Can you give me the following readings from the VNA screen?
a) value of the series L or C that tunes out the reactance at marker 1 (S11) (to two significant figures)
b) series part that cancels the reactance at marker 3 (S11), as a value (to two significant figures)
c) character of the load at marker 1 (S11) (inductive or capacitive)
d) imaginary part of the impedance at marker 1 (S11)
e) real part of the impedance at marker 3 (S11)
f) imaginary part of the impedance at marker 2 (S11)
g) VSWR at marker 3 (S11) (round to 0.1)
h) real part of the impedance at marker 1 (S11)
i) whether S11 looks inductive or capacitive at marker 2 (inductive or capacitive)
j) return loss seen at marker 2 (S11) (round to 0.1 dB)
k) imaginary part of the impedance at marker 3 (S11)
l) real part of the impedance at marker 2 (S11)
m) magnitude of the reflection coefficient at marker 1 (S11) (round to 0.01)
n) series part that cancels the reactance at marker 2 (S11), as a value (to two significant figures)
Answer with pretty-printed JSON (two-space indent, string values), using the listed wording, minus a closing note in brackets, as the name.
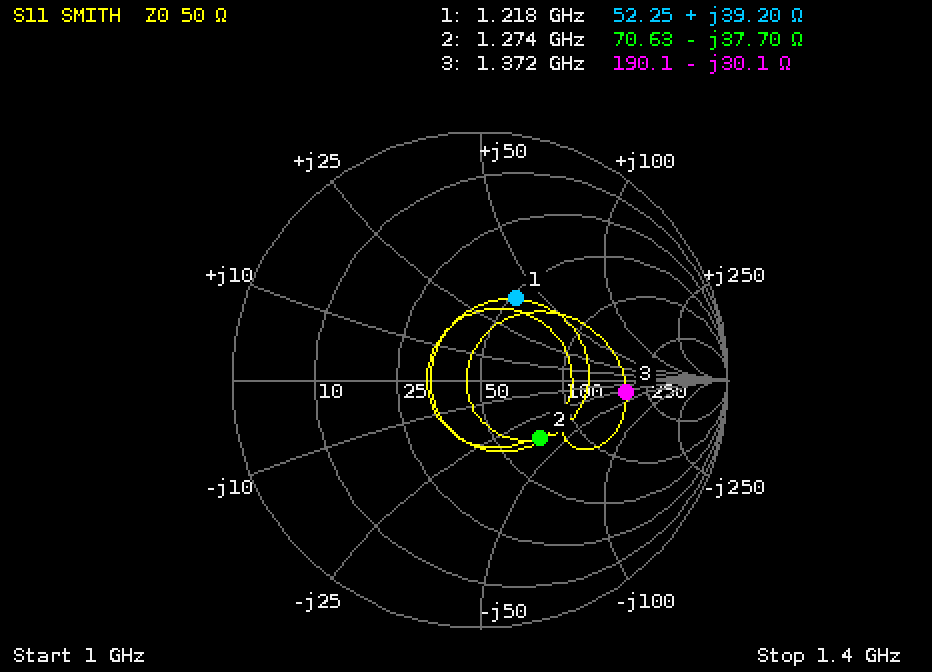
{
  "value of the series L or C that tunes out the reactance at marker 1 (S11)": "3.3 pF",
  "series part that cancels the reactance at marker 3 (S11), as a value": "3.5 nH",
  "character of the load at marker 1 (S11)": "inductive",
  "imaginary part of the impedance at marker 1": "+39.20 Ω",
  "real part of the impedance at marker 3": "190.1 Ω",
  "imaginary part of the impedance at marker 2": "-37.70 Ω",
  "VSWR at marker 3 (S11)": "3.9",
  "real part of the impedance at marker 1": "52.25 Ω",
  "whether S11 looks inductive or capacitive at marker 2": "capacitive",
  "return loss seen at marker 2 (S11)": "9.4 dB",
  "imaginary part of the impedance at marker 3": "-30.1 Ω",
  "real part of the impedance at marker 2": "70.63 Ω",
  "magnitude of the reflection coefficient at marker 1 (S11)": "0.36",
  "series part that cancels the reactance at marker 2 (S11), as a value": "4.7 nH"
}
